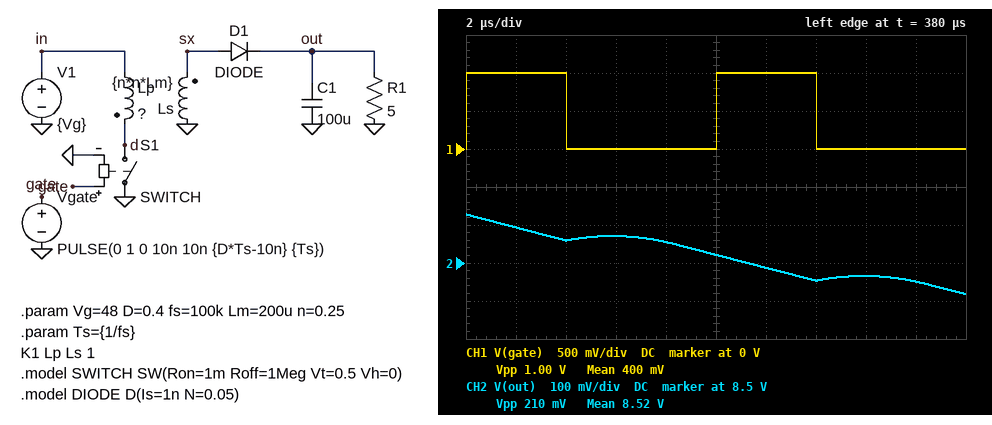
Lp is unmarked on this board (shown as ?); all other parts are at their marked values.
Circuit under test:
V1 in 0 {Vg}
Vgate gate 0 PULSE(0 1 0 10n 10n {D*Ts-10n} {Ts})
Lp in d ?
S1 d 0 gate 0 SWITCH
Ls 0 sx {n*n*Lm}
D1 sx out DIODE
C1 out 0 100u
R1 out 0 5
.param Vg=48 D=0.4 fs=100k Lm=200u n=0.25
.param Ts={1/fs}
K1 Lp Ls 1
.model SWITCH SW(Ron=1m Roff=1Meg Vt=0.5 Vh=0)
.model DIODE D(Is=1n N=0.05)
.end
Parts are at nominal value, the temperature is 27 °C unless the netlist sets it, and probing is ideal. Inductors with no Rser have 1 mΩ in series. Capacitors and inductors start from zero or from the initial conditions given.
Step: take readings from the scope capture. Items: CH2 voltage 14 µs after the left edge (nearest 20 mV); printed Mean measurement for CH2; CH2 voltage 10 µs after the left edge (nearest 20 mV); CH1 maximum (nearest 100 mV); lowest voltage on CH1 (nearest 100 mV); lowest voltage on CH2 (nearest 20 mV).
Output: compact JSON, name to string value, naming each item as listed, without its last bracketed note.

{"CH2 voltage 14 µs after the left edge": "8.46 V", "printed Mean measurement for CH2": "8.52 V", "CH2 voltage 10 µs after the left edge": "8.52 V", "CH1 maximum": "1.0 V", "lowest voltage on CH1": "0 V", "lowest voltage on CH2": "8.42 V"}
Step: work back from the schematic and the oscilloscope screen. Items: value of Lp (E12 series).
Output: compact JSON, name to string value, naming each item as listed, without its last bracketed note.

{"value of Lp": "330 µH"}
